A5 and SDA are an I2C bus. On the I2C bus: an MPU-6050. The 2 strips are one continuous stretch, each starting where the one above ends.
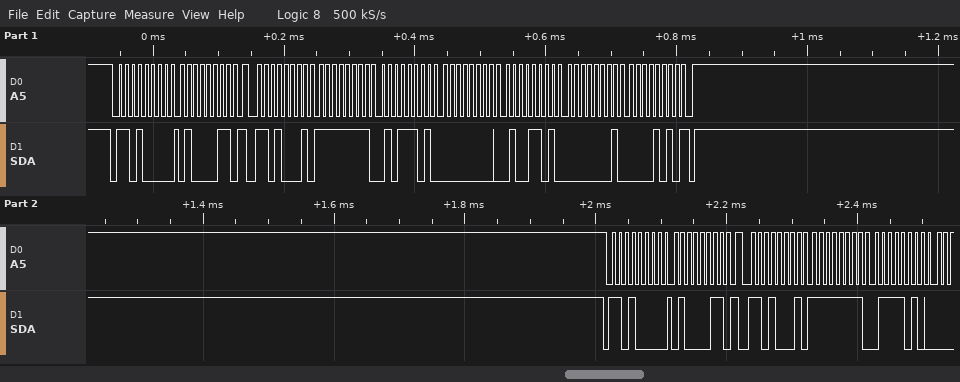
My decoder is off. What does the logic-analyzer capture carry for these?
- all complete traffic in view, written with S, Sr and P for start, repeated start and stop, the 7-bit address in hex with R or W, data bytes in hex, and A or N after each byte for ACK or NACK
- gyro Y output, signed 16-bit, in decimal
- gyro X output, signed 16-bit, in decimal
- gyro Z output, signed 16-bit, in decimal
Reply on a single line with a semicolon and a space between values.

S 68W A 43 A Sr 68R A FF A 5D A 00 A 4D A 01 A 0A N P S 68W A 43 A Sr 68R A FF A 7A A; 77; -163; 266
